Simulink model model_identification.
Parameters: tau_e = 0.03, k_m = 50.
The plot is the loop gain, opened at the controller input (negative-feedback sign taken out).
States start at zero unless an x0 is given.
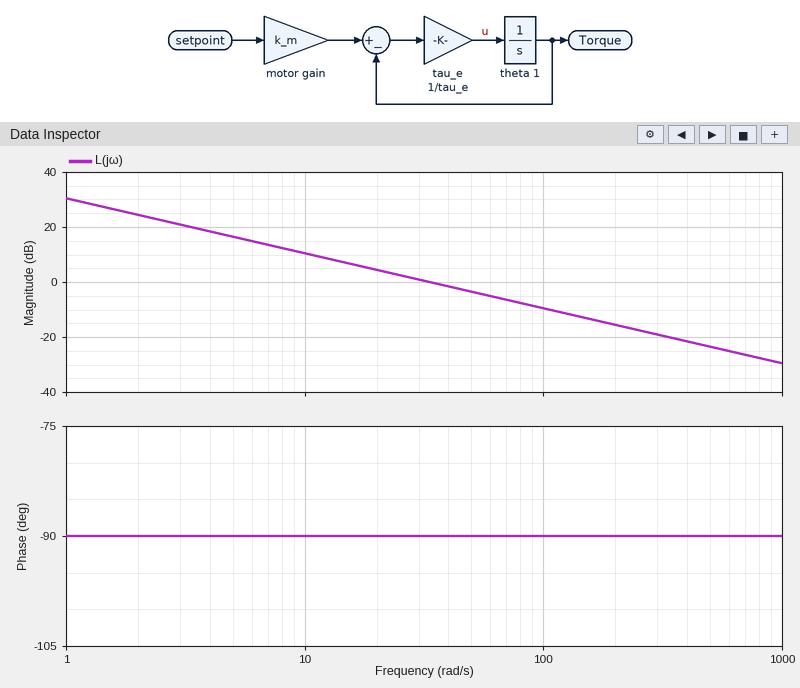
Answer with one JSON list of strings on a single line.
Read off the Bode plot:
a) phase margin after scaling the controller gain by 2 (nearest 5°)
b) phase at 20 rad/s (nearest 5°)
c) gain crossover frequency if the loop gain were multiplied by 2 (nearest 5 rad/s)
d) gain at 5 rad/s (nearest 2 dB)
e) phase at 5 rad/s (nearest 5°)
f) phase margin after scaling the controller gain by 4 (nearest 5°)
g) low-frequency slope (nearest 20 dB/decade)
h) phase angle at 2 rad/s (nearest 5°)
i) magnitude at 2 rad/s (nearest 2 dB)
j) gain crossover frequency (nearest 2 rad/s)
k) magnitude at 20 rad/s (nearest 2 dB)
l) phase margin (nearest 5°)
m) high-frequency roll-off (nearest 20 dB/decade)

["90°", "-90°", "65 rad/s", "16 dB", "-90°", "90°", "-20 dB/decade", "-90°", "24 dB", "34 rad/s", "4 dB", "90°", "-20 dB/decade"]
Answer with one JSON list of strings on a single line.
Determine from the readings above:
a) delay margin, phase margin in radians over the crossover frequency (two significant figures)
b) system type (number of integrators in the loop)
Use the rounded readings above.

["0.046 s", "1"]
